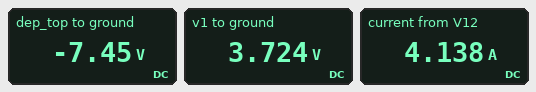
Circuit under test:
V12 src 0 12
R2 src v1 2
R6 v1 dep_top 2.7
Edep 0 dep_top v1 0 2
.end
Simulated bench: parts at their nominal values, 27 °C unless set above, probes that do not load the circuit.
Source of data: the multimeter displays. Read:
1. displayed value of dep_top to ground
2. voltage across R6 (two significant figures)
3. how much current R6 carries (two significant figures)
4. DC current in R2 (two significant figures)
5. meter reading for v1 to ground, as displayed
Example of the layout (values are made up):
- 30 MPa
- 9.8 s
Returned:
- -7.45 V
- 11 V
- 4.1 A
- 4.1 A
- 3.724 V
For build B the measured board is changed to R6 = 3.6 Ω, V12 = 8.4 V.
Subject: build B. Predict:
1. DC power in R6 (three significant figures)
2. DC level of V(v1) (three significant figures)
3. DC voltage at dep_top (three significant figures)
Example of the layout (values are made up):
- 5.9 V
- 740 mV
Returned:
- 24.8 W
- 3.15 V
- -6.30 V
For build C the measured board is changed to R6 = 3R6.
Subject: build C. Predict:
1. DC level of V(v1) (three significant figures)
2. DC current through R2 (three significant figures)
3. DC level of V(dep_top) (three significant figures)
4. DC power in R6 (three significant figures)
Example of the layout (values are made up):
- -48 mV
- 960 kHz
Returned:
- 4.50 V
- 3.75 A
- -9.00 V
- 50.6 W
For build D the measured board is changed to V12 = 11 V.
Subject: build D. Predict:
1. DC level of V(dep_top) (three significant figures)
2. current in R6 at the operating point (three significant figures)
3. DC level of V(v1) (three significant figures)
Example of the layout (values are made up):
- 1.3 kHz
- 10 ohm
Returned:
- -6.83 V
- 3.79 A
- 3.41 V
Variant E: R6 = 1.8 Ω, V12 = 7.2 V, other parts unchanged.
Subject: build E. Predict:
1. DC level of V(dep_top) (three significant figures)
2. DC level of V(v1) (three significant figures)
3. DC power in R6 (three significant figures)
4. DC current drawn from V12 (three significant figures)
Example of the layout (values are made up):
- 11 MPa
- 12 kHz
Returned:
- -3.32 V
- 1.66 V
- 13.8 W
- 2.77 A
